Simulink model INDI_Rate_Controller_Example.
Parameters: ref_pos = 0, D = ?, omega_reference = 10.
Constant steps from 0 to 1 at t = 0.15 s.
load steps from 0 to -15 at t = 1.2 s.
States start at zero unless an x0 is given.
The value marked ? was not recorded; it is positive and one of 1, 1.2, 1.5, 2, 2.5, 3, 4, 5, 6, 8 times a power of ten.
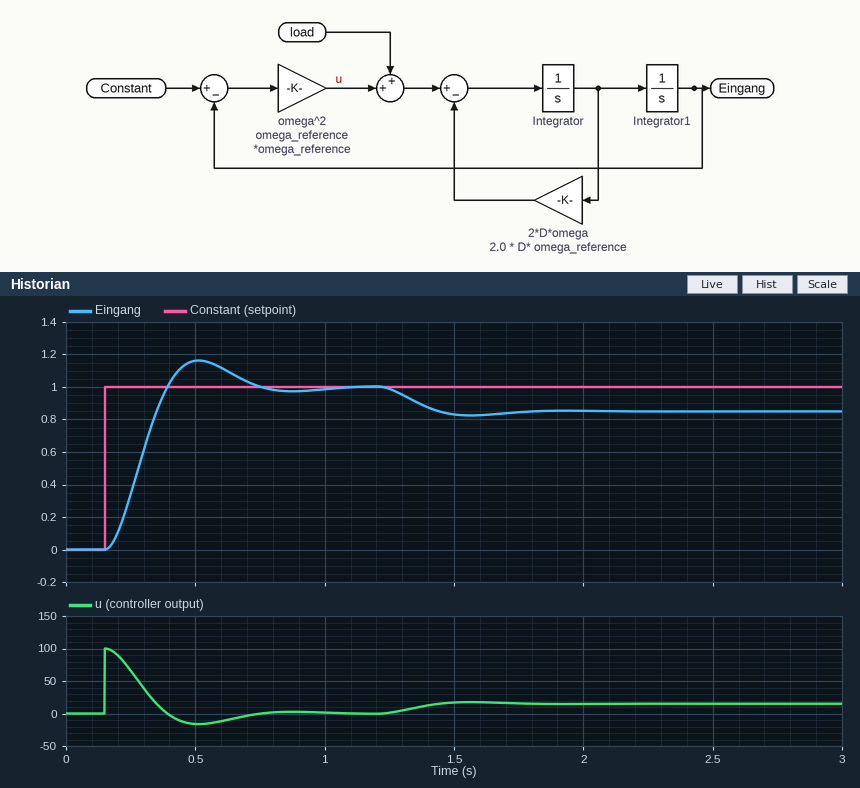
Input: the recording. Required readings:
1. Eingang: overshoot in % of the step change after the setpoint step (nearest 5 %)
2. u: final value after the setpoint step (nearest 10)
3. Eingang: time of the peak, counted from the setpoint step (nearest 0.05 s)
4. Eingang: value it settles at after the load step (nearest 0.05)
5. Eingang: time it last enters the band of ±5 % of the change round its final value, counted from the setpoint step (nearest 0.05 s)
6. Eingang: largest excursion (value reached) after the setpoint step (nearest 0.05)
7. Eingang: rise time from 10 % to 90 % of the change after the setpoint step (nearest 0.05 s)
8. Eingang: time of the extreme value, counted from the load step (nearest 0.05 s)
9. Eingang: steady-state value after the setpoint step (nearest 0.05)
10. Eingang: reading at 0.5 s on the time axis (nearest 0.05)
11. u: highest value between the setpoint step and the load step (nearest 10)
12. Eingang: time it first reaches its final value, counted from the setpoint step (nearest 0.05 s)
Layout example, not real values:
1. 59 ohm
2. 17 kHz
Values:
1. 15 %
2. 0
3. 0.35 s
4. 0.85
5. 0.55 s
6. 1.15
7. 0.15 s
8. 0.35 s
9. 1.00
10. 1.15
11. 100
12. 0.25 s
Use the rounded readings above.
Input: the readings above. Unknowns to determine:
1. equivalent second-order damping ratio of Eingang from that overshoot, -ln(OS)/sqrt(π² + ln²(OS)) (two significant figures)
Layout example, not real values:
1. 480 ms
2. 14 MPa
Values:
1. 0.52
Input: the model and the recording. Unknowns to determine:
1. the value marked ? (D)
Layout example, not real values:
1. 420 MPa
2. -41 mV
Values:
1. 0.5
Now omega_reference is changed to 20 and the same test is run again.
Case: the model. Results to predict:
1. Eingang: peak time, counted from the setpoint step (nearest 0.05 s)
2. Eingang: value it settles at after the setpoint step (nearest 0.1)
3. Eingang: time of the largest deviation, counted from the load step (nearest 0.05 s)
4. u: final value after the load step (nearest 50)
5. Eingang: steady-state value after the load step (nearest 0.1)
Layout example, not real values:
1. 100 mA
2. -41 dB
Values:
1. 0.20 s
2. 1.0
3. 0.20 s
4. 0
5. 1.0
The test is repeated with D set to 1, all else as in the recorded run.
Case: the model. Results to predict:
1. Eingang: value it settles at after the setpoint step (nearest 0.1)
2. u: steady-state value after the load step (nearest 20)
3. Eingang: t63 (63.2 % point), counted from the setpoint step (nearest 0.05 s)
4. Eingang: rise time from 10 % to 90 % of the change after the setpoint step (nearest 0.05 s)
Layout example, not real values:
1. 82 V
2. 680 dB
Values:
1. 1.0
2. 20
3. 0.20 s
4. 0.35 s
